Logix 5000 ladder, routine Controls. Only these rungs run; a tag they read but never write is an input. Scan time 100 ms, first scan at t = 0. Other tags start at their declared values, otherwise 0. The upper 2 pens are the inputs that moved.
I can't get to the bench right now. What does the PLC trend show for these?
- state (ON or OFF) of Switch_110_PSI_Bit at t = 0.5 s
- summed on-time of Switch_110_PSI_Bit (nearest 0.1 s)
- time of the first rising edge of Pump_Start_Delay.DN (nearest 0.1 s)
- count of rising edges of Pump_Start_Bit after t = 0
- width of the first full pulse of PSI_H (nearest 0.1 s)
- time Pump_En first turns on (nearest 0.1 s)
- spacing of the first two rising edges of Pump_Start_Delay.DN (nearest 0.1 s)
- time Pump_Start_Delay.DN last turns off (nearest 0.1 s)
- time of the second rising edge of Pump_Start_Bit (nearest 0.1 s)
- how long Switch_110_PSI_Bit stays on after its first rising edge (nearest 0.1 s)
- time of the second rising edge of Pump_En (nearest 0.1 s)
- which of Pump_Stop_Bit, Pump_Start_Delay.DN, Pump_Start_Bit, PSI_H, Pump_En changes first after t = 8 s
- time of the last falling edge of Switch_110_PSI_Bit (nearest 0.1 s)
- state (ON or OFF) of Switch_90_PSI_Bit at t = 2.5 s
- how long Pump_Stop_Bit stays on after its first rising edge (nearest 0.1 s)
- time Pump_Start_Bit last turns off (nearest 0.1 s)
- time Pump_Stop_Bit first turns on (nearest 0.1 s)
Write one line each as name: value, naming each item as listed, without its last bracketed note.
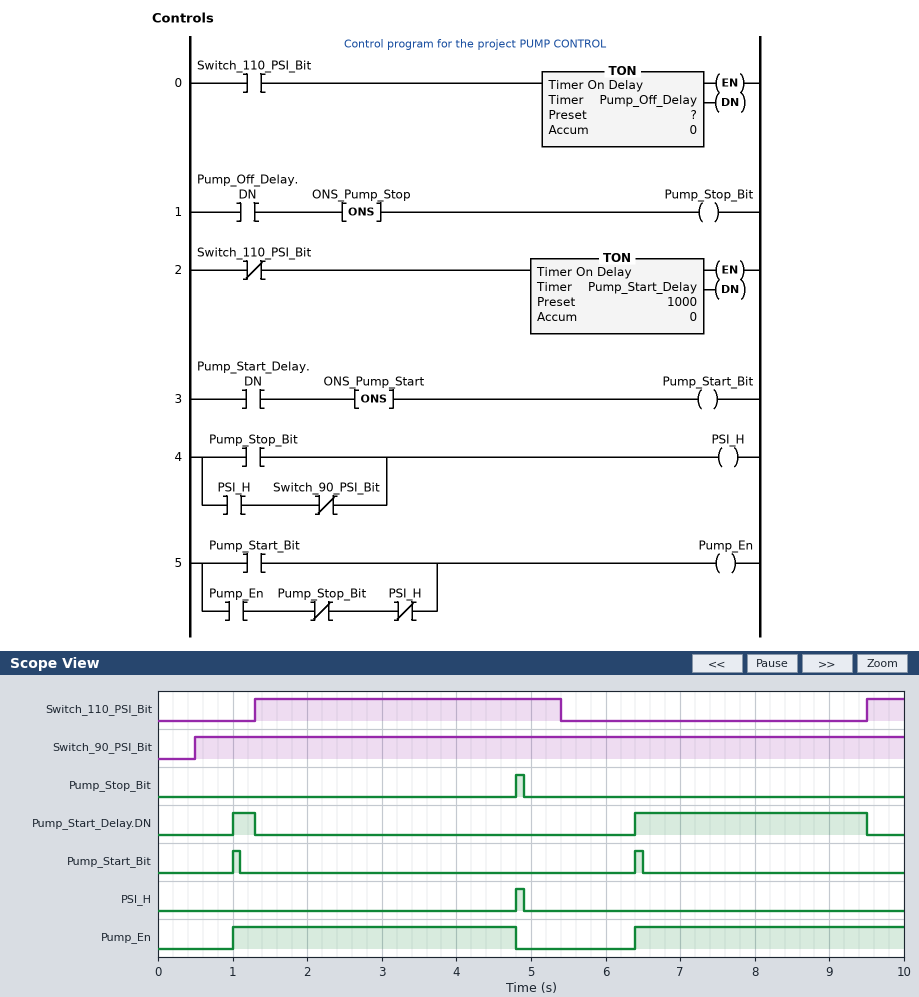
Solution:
state (ON or OFF) of Switch_110_PSI_Bit at t = 0.5 s: OFF
summed on-time of Switch_110_PSI_Bit: 4.6 s
time of the first rising edge of Pump_Start_Delay.DN: 1.0 s
count of rising edges of Pump_Start_Bit after t = 0: 2
width of the first full pulse of PSI_H: 0.1 s
time Pump_En first turns on: 1.0 s
spacing of the first two rising edges of Pump_Start_Delay.DN: 5.4 s
time Pump_Start_Delay.DN last turns off: 9.5 s
time of the second rising edge of Pump_Start_Bit: 6.4 s
how long Switch_110_PSI_Bit stays on after its first rising edge: 4.1 s
time of the second rising edge of Pump_En: 6.4 s
which of Pump_Stop_Bit, Pump_Start_Delay.DN, Pump_Start_Bit, PSI_H, Pump_En changes first after t = 8 s: Pump_Start_Delay.DN
time of the last falling edge of Switch_110_PSI_Bit: 5.4 s
state (ON or OFF) of Switch_90_PSI_Bit at t = 2.5 s: ON
how long Pump_Stop_Bit stays on after its first rising edge: 0.1 s
time Pump_Start_Bit last turns off: 6.5 s
time Pump_Stop_Bit first turns on: 4.8 s
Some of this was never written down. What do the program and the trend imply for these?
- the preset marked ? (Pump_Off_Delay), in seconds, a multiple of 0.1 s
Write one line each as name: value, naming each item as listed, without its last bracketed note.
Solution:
the preset marked ? (Pump_Off_Delay), in seconds, a multiple of 0.1 s: 3.5 s
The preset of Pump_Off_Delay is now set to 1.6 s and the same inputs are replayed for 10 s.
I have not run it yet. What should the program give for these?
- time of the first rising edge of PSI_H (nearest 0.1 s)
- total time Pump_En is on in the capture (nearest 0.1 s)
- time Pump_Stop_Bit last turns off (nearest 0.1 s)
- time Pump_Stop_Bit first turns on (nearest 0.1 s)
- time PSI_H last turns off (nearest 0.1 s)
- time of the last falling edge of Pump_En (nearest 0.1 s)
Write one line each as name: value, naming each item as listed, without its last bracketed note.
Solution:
time of the first rising edge of PSI_H: 2.9 s
total time Pump_En is on in the capture: 5.5 s
time Pump_Stop_Bit last turns off: 3.0 s
time Pump_Stop_Bit first turns on: 2.9 s
time PSI_H last turns off: 3.0 s
time of the last falling edge of Pump_En: 2.9 s
